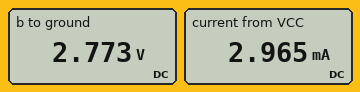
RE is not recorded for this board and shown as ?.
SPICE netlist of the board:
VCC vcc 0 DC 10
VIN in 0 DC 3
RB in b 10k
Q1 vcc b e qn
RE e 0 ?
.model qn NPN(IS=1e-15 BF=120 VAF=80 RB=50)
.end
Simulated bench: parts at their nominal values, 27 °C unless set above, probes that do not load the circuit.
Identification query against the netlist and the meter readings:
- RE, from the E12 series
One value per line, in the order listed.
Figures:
680 Ω
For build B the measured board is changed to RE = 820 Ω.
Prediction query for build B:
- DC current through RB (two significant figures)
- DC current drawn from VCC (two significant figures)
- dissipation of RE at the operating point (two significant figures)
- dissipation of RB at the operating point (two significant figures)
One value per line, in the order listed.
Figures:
19 µA
2.5 mA
5.2 mW
3.7 µW
